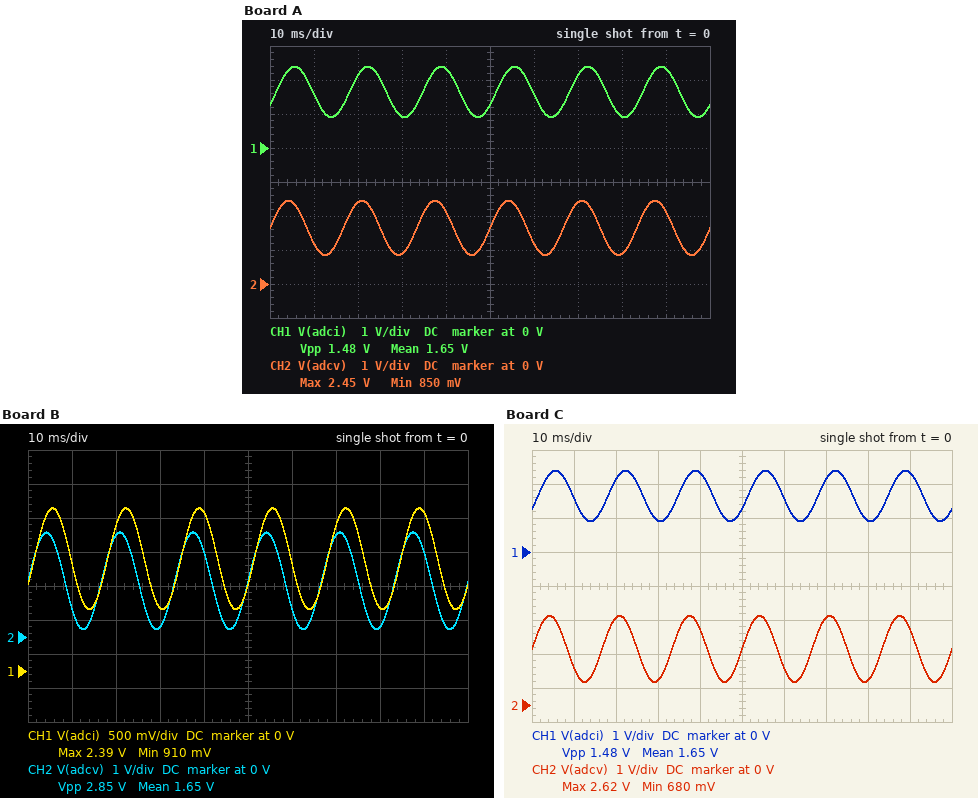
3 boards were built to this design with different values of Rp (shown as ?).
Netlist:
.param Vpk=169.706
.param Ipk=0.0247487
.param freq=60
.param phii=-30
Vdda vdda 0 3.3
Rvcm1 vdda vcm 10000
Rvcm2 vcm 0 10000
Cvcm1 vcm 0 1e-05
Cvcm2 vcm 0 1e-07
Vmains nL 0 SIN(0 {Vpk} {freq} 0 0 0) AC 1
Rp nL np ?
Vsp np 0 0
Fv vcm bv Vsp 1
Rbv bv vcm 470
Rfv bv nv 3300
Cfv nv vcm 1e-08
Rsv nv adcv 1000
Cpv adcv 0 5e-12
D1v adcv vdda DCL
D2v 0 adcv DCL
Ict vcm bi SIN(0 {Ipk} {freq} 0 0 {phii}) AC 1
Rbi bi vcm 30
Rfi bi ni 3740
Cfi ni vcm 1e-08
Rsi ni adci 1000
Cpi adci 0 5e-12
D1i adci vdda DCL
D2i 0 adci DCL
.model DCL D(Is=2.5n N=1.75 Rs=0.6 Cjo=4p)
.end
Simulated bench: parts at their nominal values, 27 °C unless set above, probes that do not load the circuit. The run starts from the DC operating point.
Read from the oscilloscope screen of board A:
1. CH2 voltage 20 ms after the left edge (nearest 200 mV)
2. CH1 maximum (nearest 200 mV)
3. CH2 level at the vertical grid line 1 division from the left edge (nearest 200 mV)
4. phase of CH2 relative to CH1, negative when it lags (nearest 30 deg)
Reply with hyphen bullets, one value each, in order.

- 2.4 V
- 2.4 V
- 1.2 V
- 30 deg
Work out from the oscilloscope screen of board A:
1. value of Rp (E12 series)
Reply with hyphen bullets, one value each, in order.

- 100 kΩ
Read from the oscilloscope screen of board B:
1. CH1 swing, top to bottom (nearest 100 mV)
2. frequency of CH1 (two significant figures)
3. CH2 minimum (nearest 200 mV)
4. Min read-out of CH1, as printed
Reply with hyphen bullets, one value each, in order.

- 1.5 V
- 60 Hz
- 200 mV
- 910 mV
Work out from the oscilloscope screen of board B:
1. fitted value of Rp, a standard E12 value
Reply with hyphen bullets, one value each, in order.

- 56 kΩ
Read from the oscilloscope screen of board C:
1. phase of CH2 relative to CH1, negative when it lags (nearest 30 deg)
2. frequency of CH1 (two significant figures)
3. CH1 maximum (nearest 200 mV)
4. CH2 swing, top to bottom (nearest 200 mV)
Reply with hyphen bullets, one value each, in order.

- 30 deg
- 60 Hz
- 2.4 V
- 2.0 V
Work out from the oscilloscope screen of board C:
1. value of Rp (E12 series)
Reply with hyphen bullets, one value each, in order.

- 82 kΩ
